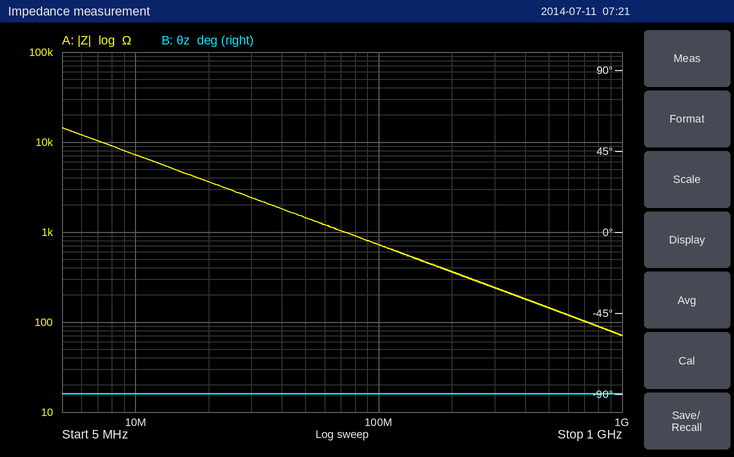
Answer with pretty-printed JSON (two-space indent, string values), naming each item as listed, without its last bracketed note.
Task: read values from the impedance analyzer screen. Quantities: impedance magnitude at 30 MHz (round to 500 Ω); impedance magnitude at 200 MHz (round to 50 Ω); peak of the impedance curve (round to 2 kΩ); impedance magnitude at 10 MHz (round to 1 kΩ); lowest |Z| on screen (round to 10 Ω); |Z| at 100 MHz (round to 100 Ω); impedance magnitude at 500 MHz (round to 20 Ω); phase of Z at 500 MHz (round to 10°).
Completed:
{
  "impedance magnitude at 30 MHz": "2.5 kΩ",
  "impedance magnitude at 200 MHz": "350 Ω",
  "peak of the impedance curve": "14 kΩ",
  "impedance magnitude at 10 MHz": "7 kΩ",
  "lowest |Z| on screen": "70 Ω",
  "|Z| at 100 MHz": "700 Ω",
  "impedance magnitude at 500 MHz": "140 Ω",
  "phase of Z at 500 MHz": "-90°"
}
